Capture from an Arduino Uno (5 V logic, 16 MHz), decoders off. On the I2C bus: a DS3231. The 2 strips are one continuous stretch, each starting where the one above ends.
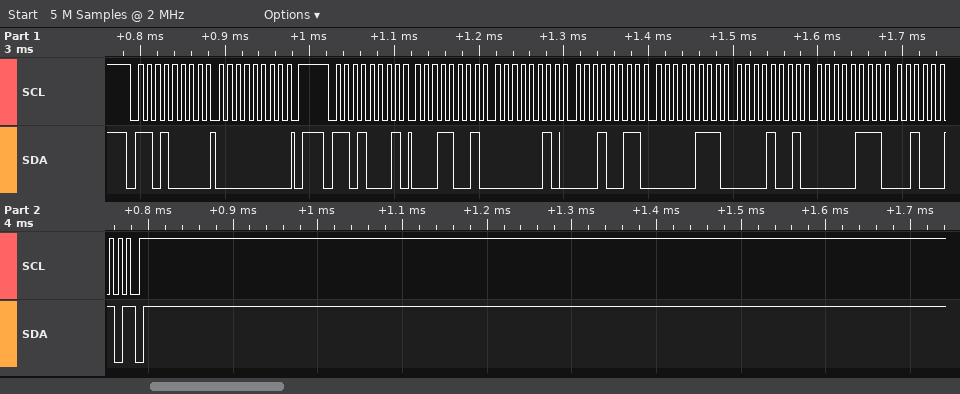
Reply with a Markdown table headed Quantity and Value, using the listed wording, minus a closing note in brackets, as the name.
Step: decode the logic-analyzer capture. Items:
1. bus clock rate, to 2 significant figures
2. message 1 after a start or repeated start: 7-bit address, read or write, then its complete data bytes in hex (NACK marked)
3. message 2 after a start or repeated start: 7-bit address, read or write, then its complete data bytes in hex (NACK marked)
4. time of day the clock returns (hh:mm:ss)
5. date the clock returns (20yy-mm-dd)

| Quantity | Value |
|---|---|
| bus clock rate, to 2 significant figures | 100 kHz |
| message 1 after a start or repeated start: 7-bit address, read or write, then its complete data bytes in hex | 0x68 write: 00 |
| message 2 after a start or repeated start: 7-bit address, read or write, then its complete data bytes in hex | 0x68 read: 19 02 13 07 09 07 22 NACK |
| time of day the clock returns | 13:02:19 |
| date the clock returns | 2022-07-09 |
